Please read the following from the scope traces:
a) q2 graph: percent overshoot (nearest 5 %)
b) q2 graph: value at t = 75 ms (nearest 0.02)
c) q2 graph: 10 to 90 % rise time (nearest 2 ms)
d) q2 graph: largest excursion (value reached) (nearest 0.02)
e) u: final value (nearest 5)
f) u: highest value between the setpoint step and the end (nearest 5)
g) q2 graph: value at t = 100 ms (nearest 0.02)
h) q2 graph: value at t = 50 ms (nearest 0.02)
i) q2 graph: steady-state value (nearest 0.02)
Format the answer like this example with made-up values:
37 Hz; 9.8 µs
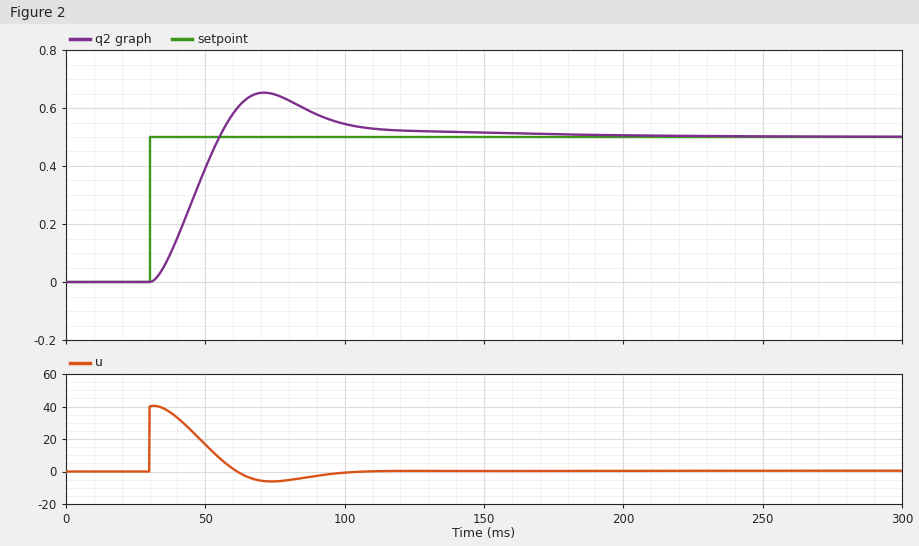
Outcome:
30 %; 0.64; 18 ms; 0.66; 0; 40; 0.54; 0.40; 0.50
